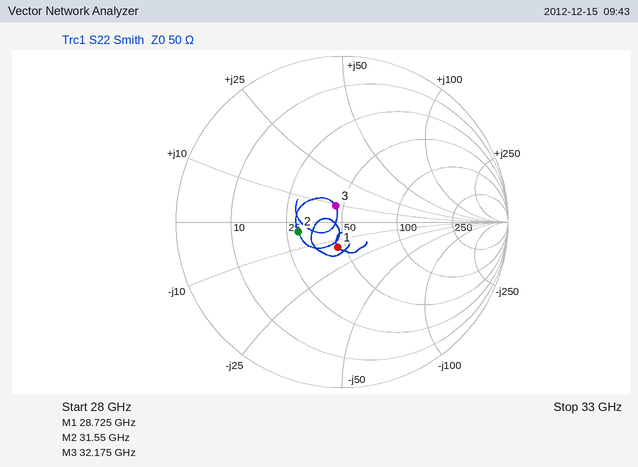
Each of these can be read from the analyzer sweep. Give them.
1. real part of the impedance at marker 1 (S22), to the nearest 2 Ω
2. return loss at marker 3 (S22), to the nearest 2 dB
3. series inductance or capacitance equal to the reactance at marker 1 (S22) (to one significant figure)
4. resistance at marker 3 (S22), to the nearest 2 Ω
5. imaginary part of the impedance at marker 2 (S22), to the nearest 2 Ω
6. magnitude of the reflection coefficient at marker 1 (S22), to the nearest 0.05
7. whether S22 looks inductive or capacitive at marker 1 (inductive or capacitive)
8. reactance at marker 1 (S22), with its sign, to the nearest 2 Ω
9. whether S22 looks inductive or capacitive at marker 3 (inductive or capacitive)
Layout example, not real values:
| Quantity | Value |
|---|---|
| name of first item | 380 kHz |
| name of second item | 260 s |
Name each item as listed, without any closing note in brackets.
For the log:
| Quantity | Value |
|---|---|
| real part of the impedance at marker 1 (S22), to the nearest 2 Ω | 46 Ω |
| return loss at marker 3 (S22), to the nearest 2 dB | 20 dB |
| series inductance or capacitance equal to the reactance at marker 1 (S22) | 400 fF |
| resistance at marker 3 (S22), to the nearest 2 Ω | 46 Ω |
| imaginary part of the impedance at marker 2 (S22), to the nearest 2 Ω | -4 Ω |
| magnitude of the reflection coefficient at marker 1 (S22), to the nearest 0.05 | 0.15 |
| whether S22 looks inductive or capacitive at marker 1 | capacitive |
| reactance at marker 1 (S22), with its sign, to the nearest 2 Ω | -14 Ω |
| whether S22 looks inductive or capacitive at marker 3 | inductive |
